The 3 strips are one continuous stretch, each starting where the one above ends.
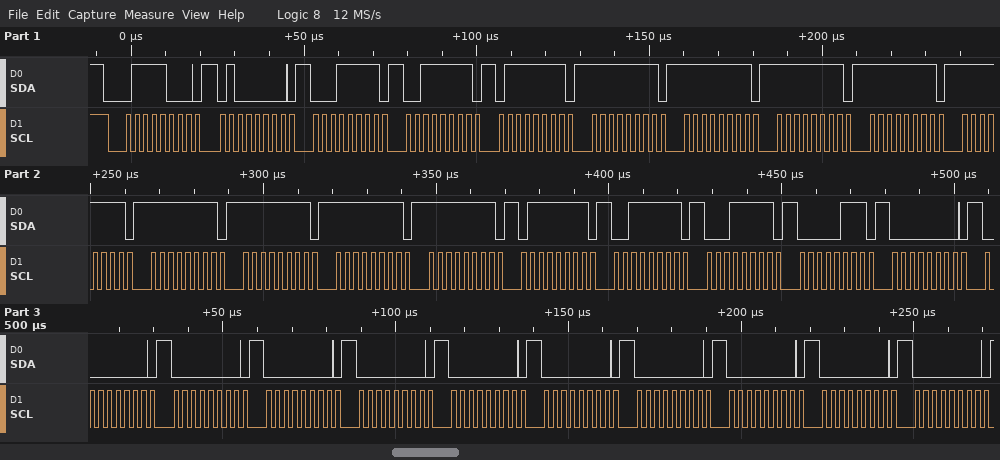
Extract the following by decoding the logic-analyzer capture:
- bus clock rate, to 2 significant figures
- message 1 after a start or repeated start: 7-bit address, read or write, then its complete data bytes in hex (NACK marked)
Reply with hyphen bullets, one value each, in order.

- 400 kHz
- 0x3C write: 40 1F 3F 7F FF FF FF FF FF FF FF FF FF 7F 3F 1F 07 00 00 00 00 00 00 00 00 00 00 00
